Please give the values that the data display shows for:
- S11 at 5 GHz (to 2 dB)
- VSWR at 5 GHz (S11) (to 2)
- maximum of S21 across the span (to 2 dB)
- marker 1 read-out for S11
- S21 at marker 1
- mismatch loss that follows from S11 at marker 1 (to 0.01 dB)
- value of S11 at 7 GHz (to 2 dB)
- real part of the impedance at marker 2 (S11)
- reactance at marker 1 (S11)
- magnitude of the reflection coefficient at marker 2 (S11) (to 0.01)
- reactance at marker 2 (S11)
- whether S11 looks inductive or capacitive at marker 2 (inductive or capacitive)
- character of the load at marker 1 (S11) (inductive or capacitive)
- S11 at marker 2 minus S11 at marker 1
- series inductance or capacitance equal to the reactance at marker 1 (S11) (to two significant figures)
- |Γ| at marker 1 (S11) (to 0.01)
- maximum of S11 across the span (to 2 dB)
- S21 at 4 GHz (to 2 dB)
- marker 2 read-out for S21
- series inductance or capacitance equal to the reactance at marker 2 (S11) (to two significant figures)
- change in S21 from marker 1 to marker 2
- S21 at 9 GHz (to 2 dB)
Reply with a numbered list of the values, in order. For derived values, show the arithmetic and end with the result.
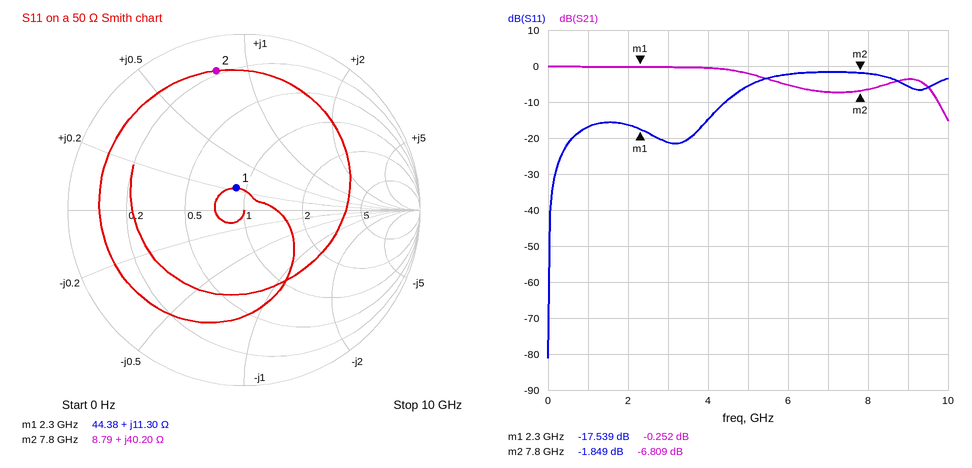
1. -6 dB
2. |Γ| = 10^(-6/20) = 0.5012; VSWR = (1 + 0.5012)/(1 − 0.5012) ≈ 3.01, so 4 to the nearest 2
3. 0 dB
4. -17.539 dB
5. -0.252 dB
6. −10 log10(1 − 10^(-17.539/10)) ≈ 0.08 dB
7. -2 dB
8. 8.79 Ω
9. +11.30 Ω
10. 0.81
11. +40.20 Ω
12. inductive
13. inductive
14. -1.849 − (-17.539) = 15.690 dB
15. L = 11.3 Ω/(2π × 2.3 GHz) ≈ 782 pH, so 780 pH to two significant figures
16. 0.13
17. -2 dB
18. 0 dB
19. -6.809 dB
20. L = 40.2 Ω/(2π × 7.8 GHz) ≈ 820 pH
21. -6.809 − (-0.252) = -6.557 dB
22. -4 dB
